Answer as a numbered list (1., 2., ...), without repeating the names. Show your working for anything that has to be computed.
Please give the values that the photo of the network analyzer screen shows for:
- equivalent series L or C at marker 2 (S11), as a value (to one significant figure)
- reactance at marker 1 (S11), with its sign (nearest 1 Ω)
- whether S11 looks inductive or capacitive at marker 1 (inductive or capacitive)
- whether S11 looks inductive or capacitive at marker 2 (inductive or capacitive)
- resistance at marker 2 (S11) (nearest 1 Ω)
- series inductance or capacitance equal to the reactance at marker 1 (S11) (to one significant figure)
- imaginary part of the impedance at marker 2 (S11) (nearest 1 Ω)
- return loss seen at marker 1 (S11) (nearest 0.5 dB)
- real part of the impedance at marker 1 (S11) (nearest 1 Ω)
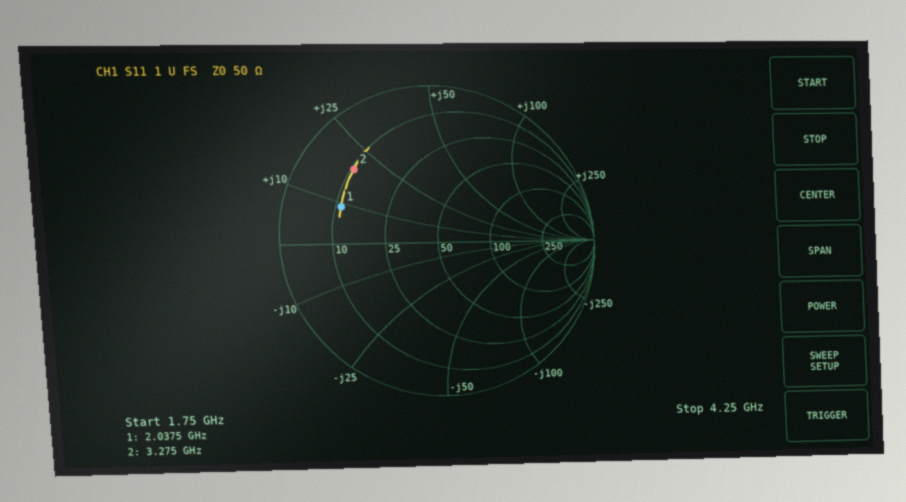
1. L = 19 Ω/(2π × 3.275 GHz) ≈ 923 pH, so 900 pH to one significant figure
2. +9 Ω
3. inductive
4. inductive
5. 11 Ω
6. L = 9 Ω/(2π × 2.0375 GHz) ≈ 703 pH, so 700 pH to one significant figure
7. +19 Ω
8. 4.0 dB
9. 11 Ω
